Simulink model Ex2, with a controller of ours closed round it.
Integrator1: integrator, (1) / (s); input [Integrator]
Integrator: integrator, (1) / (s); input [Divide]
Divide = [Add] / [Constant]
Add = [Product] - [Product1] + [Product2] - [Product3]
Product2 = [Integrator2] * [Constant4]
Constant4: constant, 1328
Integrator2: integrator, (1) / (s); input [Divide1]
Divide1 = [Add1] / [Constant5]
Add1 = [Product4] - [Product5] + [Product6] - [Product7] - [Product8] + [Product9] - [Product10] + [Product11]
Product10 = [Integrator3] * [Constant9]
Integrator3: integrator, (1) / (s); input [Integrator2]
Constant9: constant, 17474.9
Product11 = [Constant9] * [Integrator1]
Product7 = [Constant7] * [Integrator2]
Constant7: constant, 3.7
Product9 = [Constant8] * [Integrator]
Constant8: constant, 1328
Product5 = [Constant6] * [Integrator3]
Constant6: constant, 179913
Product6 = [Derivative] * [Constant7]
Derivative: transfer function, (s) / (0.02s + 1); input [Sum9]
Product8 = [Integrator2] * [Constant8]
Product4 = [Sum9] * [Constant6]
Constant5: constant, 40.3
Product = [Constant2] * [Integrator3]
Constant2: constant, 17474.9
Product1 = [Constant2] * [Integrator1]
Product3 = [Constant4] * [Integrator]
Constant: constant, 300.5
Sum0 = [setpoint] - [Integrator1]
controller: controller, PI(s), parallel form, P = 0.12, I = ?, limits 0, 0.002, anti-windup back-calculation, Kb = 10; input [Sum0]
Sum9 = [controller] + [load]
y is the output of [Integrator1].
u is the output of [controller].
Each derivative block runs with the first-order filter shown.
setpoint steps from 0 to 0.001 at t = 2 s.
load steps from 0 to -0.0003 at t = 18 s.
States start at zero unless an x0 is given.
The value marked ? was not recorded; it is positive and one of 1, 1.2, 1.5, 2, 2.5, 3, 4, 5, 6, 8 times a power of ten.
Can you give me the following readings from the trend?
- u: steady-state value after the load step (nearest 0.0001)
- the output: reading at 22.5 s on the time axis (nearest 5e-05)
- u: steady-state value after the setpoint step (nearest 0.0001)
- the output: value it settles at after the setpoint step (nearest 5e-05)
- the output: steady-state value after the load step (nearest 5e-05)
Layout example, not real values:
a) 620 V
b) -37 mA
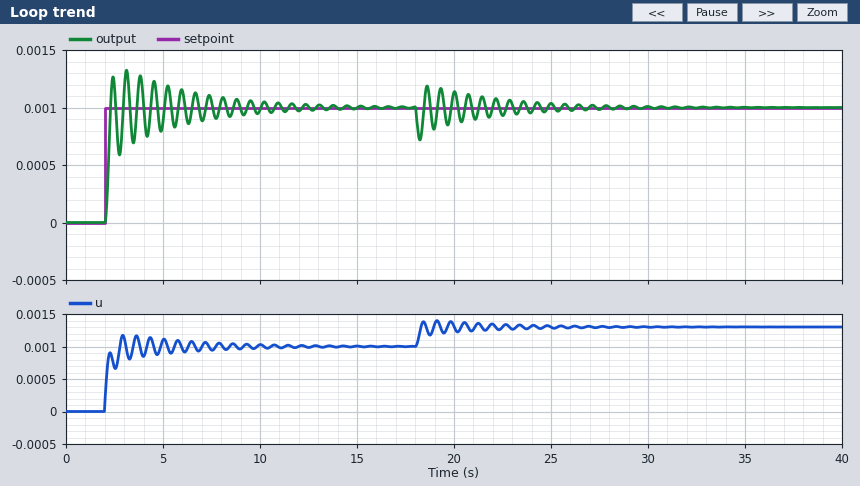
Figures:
a) 0.0013
b) 0.00095
c) 0.0010
d) 0.00100
e) 0.00100
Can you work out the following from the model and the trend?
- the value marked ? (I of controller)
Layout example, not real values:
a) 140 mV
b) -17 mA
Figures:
a) 5
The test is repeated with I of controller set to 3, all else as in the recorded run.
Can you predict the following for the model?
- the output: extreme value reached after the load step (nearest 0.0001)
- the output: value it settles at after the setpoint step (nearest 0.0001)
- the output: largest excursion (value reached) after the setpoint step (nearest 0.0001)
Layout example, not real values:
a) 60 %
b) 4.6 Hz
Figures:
a) 0.0007
b) 0.0010
c) 0.0011
